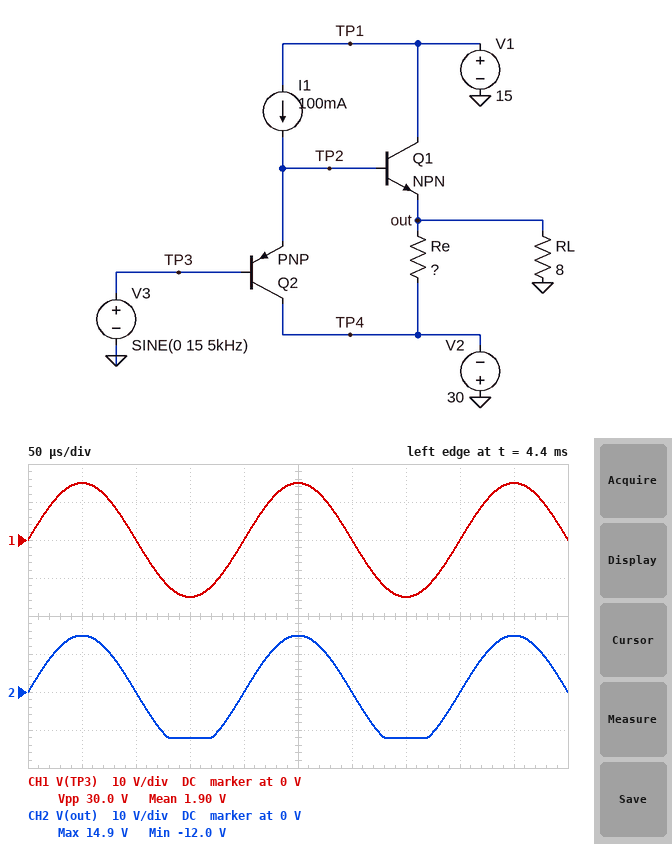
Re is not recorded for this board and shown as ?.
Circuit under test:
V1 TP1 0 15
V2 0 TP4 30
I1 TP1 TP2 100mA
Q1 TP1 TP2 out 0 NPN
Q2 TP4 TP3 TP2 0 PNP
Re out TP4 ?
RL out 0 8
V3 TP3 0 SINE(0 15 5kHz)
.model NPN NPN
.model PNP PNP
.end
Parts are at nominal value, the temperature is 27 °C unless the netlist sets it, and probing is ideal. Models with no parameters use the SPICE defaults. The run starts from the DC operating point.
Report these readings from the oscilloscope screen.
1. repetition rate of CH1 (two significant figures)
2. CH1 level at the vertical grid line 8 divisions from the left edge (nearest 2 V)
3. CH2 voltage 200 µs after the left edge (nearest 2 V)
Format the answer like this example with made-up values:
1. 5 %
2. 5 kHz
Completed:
1. 5.0 kHz
2. 0 V
3. 0 V
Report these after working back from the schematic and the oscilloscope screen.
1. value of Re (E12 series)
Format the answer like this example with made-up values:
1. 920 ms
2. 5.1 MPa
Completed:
1. 12 Ω
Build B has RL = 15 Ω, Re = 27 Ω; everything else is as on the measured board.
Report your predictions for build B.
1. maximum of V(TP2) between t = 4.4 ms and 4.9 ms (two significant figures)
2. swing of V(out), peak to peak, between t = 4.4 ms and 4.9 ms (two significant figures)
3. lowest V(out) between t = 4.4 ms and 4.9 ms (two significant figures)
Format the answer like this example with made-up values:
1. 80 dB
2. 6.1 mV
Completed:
1. 16 V
2. 26 V
3. -11 V
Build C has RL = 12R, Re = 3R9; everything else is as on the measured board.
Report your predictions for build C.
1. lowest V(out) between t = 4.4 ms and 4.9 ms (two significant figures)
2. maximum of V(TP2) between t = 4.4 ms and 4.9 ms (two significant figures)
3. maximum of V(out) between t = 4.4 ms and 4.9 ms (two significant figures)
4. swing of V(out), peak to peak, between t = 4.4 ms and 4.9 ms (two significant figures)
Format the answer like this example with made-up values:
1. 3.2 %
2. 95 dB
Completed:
1. -15 V
2. 8.1 V
3. 7.1 V
4. 22 V
